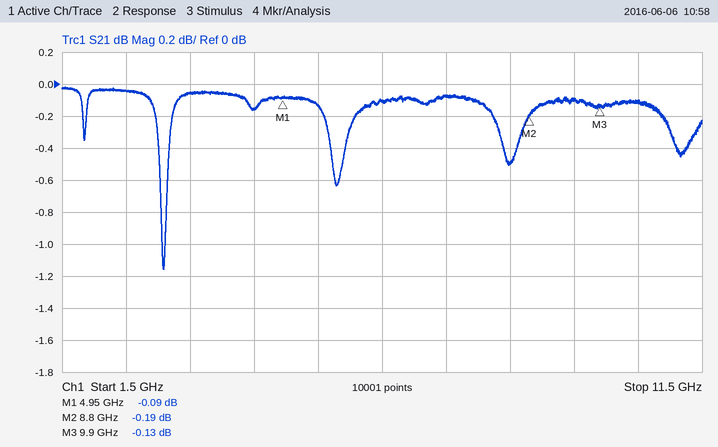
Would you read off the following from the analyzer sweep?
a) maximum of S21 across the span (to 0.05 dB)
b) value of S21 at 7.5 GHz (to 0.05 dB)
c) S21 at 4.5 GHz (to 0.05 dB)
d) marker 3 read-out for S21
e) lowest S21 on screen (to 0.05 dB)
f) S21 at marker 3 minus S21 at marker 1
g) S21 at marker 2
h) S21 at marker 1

0.00 dB
-0.10 dB
-0.15 dB
-0.13 dB
-1.15 dB
-0.04 dB
-0.19 dB
-0.09 dB
